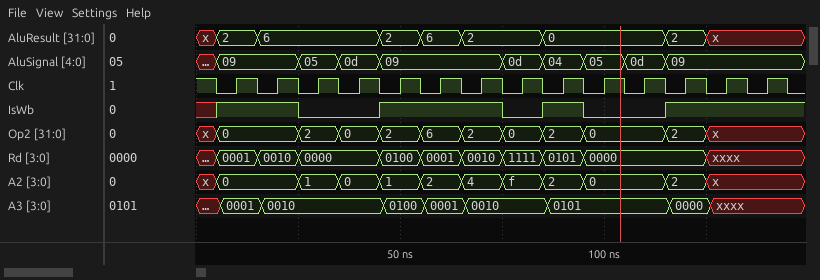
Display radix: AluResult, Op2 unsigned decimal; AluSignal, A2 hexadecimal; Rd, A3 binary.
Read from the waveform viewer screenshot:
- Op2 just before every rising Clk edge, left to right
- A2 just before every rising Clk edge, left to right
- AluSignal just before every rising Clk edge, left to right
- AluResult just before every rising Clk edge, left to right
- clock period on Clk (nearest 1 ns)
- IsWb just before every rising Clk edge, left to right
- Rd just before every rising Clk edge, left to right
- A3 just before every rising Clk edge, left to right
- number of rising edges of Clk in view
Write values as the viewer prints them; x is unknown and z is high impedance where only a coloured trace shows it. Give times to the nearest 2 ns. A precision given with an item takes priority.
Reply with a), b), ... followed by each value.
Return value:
a) 0, 0, 2, 0, 2, 6, 2, 0, 2, 0, 0, 2, x, x
b) 0, 0, 1, 0, 1, 2, 4, f, 2, 0, 0, 2, x, x
c) 09, 09, 05, 0d, 09, 09, 09, 0d, 04, 05, 0d, 09, 09, 09
d) 2, 6, 6, 6, 2, 6, 2, 2, 0, 0, 0, 2, x, x
e) 10 ns
f) 1 1 0 0 1 1 1 0 1 0 0 1 1 1
g) 0001, 0010, 0000, 0000, 0100, 0001, 0010, 1111, 0101, 0000, 0000, 0000, xxxx, xxxx
h) 0001, 0010, 0010, 0010, 0100, 0001, 0010, 0010, 0101, 0101, 0101, 0000, xxxx, xxxx
i) 14
